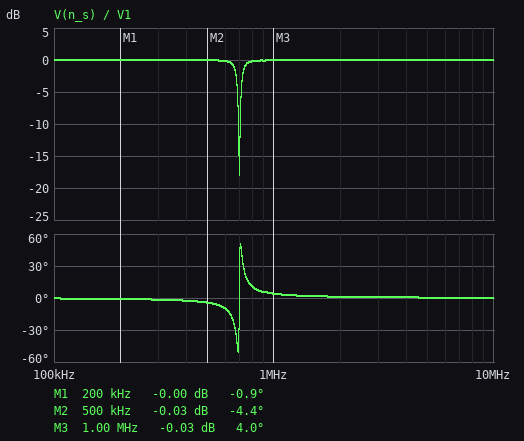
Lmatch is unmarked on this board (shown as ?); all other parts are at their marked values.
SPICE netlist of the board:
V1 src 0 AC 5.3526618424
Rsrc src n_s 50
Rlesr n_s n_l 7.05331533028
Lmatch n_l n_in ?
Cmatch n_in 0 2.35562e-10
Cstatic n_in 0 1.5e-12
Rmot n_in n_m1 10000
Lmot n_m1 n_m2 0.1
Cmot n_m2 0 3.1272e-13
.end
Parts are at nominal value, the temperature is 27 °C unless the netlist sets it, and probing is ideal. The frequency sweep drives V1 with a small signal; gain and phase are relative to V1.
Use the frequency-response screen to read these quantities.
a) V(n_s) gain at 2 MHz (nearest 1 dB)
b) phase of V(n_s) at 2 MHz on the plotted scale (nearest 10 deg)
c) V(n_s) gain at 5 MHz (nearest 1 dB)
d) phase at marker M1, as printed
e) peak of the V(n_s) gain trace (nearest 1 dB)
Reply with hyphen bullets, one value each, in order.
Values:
- 0 dB
- 0 deg
- 0 dB
- -0.9 deg
- 0 dB
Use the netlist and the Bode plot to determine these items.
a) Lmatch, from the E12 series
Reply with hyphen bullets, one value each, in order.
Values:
- 220 µH
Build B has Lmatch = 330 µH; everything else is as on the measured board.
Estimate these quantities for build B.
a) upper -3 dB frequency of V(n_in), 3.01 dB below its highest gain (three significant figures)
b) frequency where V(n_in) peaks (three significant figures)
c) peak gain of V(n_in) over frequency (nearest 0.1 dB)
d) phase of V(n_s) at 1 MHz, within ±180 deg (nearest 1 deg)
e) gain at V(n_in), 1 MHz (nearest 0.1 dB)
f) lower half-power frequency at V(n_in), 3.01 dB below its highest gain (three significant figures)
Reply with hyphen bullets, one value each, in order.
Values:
- 582 kHz
- 568 kHz
- 26.3 dB
- 2 deg
- -6.3 dB
- 554 kHz
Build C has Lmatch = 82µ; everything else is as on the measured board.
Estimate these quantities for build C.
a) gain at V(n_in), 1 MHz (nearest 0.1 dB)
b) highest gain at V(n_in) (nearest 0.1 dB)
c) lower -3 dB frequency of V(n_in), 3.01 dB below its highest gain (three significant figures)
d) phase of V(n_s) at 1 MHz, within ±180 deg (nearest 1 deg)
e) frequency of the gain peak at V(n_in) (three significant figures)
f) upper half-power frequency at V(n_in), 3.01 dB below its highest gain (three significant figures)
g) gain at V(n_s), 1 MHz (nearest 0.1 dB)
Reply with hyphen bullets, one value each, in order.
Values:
- 12.0 dB
- 20.3 dB
- 1.08 MHz
- -17 deg
- 1.14 MHz
- 1.19 MHz
- -0.5 dB
